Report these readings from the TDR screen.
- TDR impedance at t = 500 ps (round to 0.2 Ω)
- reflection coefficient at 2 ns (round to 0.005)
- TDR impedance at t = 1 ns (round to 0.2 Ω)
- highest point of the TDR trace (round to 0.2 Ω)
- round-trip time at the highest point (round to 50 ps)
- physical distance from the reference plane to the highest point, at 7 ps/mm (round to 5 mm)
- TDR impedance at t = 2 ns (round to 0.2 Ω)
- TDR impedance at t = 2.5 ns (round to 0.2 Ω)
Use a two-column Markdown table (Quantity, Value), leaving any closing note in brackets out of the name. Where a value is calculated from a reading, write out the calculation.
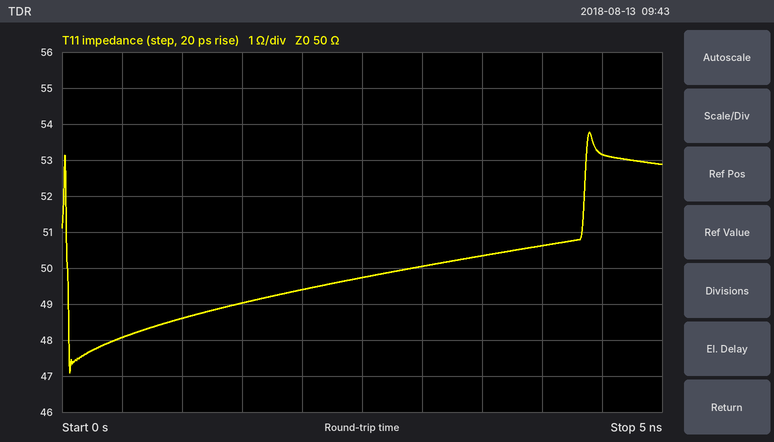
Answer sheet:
| Quantity | Value |
|---|---|
| TDR impedance at t = 500 ps | 48.0 Ω |
| reflection coefficient at 2 ns | (49.4 − 50)/(49.4 + 50) ≈ -0.00604, so -0.005 to the nearest 0.005 |
| TDR impedance at t = 1 ns | 48.6 Ω |
| highest point of the TDR trace | 53.8 Ω |
| round-trip time at the highest point | 4.40 ns |
| physical distance from the reference plane to the highest point, at 7 ps/mm | 4.40 ns / 2 / 7 ps/mm ≈ 314 mm, so 315 mm to the nearest 5 mm |
| TDR impedance at t = 2 ns | 49.4 Ω |
| TDR impedance at t = 2.5 ns | 49.8 Ω |
